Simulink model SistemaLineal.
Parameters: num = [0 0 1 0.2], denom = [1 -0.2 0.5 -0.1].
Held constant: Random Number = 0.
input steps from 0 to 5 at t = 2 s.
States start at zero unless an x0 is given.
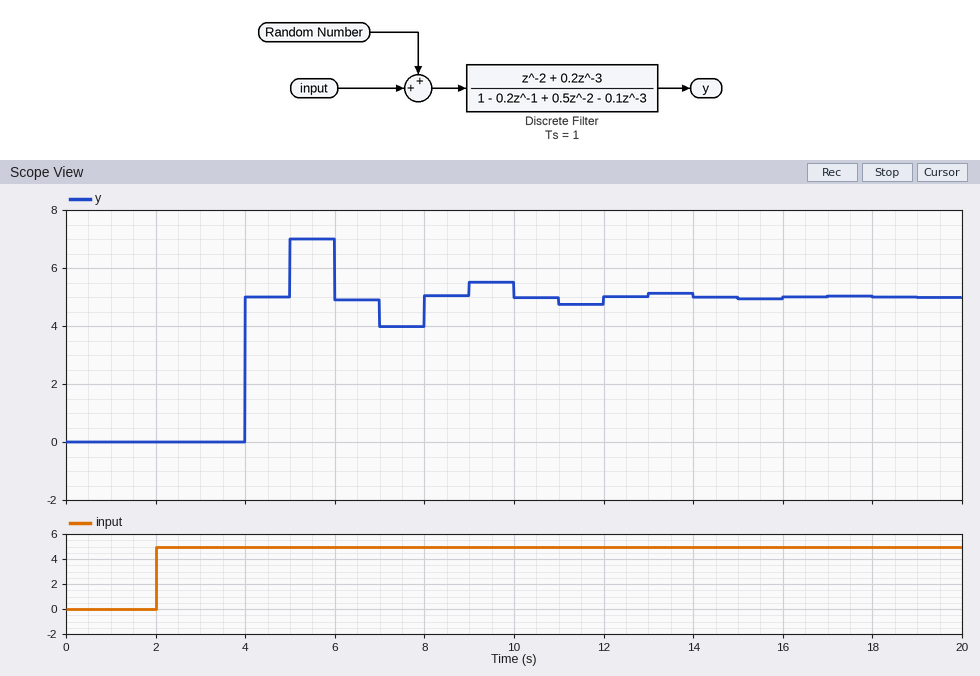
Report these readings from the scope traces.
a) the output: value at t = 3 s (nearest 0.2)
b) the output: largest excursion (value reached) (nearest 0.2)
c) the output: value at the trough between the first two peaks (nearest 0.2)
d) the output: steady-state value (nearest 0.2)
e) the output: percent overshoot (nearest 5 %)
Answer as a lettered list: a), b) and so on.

a) 0.0
b) 7.0
c) 4.0
d) 5.0
e) 40 %
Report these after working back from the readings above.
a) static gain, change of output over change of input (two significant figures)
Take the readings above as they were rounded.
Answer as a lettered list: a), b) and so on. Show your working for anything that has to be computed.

a) (5 - 0) / (5 - 0) = 1.0
